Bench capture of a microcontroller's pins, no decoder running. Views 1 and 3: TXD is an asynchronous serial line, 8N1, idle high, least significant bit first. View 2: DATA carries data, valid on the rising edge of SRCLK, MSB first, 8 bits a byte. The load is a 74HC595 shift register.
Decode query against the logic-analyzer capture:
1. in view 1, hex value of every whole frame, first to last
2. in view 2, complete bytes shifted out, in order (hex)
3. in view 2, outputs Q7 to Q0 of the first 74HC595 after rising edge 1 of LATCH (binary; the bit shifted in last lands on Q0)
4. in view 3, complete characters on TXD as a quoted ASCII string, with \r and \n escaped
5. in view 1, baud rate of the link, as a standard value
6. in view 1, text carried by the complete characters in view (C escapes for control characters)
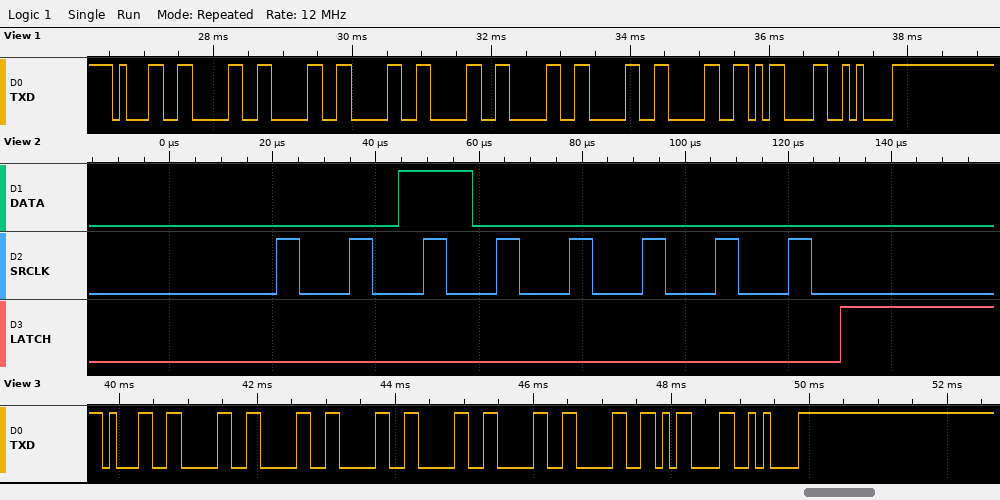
31 30 30 30 30 30 30 30 0D 0A
0x20
00100000
"1000000\r\n"
9600 baud
"10000000\r\n"
